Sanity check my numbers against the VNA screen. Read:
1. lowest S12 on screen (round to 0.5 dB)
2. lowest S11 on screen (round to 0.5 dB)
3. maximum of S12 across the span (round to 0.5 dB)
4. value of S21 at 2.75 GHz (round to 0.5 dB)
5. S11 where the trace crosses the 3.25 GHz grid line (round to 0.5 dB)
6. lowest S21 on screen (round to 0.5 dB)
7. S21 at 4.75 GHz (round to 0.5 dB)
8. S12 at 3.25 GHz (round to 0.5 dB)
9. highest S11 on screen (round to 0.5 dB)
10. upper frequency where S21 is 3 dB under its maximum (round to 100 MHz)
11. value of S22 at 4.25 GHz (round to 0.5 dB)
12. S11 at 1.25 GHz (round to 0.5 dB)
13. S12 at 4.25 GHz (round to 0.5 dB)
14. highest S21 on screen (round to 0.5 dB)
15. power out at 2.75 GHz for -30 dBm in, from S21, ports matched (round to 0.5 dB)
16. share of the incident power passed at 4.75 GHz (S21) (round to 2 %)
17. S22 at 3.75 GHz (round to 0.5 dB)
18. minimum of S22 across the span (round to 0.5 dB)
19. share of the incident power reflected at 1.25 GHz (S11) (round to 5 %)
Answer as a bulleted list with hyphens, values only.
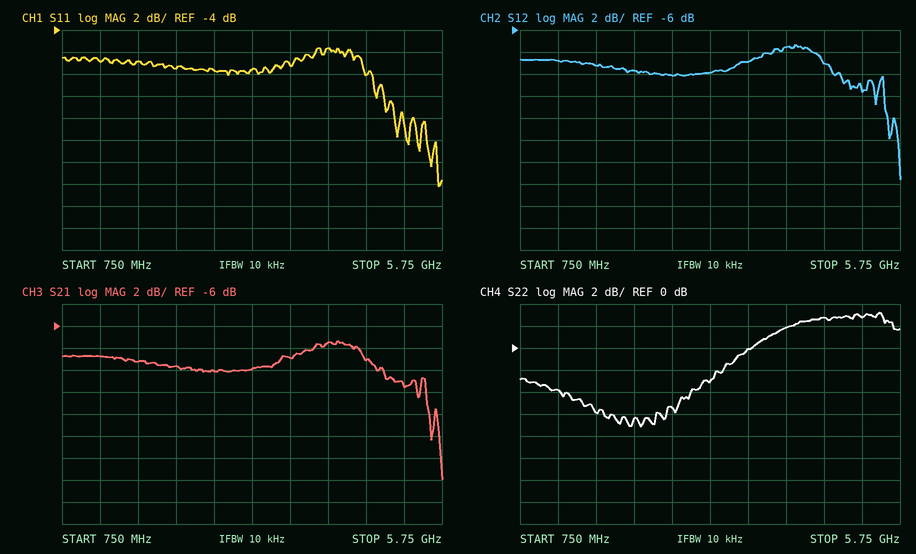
- -19.5 dB
- -18.0 dB
- -7.5 dB
- -10.0 dB
- -7.5 dB
- -20.0 dB
- -9.0 dB
- -10.0 dB
- -5.5 dB
- 5.0 GHz
- 2.0 dB
- -7.0 dB
- -7.5 dB
- -7.5 dB
- -40.0 dBm
- 12 %
- 0.0 dB
- -7.0 dB
- 20 %
